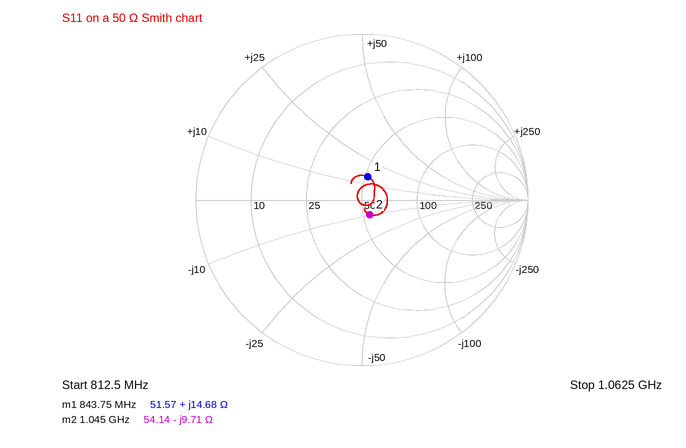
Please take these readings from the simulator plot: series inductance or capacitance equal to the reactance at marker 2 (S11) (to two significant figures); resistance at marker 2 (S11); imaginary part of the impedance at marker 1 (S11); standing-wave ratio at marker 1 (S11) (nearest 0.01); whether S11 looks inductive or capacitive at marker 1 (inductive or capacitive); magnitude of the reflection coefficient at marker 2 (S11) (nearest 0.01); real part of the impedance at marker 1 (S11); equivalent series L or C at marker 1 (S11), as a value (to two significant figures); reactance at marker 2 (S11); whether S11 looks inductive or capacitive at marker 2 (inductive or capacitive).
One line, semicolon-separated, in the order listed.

16 pF; 54.14 Ω; +14.68 Ω; 1.34; inductive; 0.10; 51.57 Ω; 2.8 nH; -9.71 Ω; capacitive
